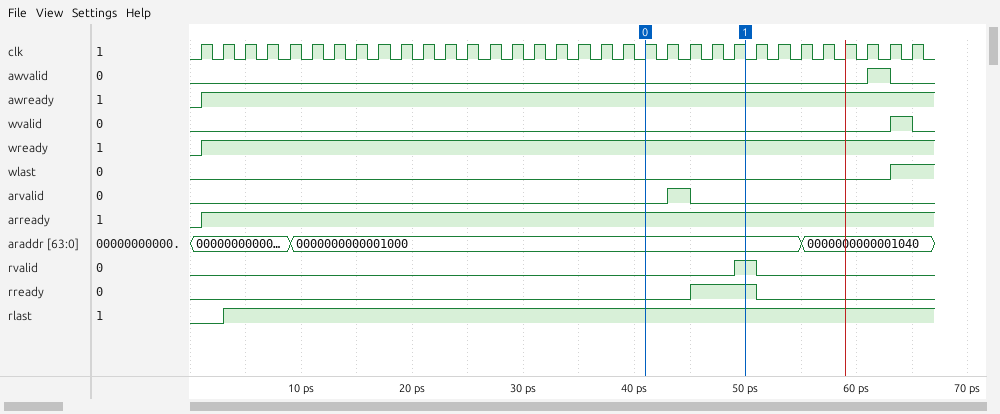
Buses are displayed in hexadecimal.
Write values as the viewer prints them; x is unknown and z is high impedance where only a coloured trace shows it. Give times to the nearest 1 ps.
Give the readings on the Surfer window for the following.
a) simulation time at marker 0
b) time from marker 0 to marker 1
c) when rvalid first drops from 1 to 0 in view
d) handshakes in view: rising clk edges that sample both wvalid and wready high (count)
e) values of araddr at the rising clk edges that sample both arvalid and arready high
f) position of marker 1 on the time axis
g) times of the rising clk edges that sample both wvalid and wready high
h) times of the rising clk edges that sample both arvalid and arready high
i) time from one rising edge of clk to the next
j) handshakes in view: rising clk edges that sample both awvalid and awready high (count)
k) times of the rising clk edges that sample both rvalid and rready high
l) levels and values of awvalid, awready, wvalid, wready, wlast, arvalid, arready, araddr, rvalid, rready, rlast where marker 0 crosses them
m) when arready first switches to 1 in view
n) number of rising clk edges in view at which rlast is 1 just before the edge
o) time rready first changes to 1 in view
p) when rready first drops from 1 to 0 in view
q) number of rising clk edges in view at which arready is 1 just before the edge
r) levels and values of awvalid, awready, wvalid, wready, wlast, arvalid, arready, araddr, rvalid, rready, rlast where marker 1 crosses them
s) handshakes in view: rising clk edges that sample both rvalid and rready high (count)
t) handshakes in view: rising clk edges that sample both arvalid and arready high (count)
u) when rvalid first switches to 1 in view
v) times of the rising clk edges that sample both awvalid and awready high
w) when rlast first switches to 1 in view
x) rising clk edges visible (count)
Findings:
41 ps
9 ps
51 ps
1
0000000000001000
50 ps
65 ps
45 ps
2 ps
1
51 ps
awvalid=0, awready=1, wvalid=0, wready=1, wlast=0, arvalid=0, arready=1, araddr=0000000000001000, rvalid=0, rready=0, rlast=1
1 ps
31
45 ps
51 ps
32
awvalid=0, awready=1, wvalid=0, wready=1, wlast=0, arvalid=0, arready=1, araddr=0000000000001000, rvalid=1, rready=1, rlast=1
1
1
49 ps
63 ps
3 ps
33
